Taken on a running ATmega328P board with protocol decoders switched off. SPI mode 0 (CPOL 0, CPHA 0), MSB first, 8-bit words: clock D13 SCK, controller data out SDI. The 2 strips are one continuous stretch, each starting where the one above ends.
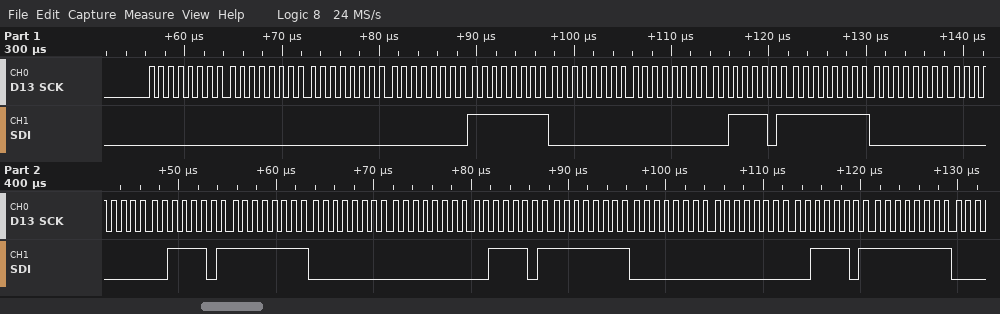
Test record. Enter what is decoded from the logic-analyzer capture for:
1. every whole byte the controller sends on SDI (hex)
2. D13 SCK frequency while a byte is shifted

00 00 00 00 FF 00 00 3D FF 00 00 3D FF 00 00 3D FF 00 00 3D FF
1 MHz
